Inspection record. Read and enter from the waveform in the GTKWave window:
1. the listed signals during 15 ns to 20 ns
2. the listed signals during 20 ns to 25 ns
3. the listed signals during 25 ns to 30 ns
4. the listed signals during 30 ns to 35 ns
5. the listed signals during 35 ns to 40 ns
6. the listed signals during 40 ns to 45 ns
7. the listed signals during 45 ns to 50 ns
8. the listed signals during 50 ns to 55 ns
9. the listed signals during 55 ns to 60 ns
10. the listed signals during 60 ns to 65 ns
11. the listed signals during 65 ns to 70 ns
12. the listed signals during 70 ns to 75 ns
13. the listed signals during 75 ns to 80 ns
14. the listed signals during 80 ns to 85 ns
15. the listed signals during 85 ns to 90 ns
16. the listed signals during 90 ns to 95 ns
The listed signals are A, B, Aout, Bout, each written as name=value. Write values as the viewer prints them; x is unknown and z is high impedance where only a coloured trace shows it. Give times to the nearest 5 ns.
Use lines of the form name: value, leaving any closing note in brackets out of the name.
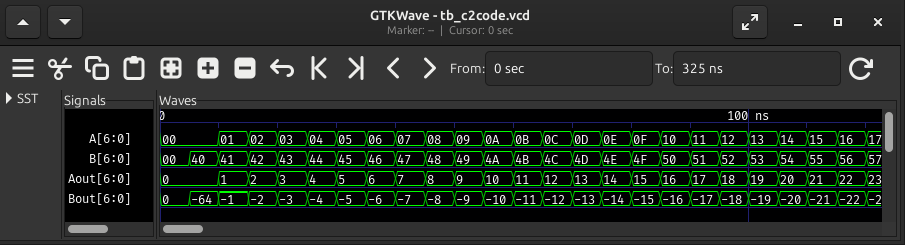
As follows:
the listed signals during 15 ns to 20 ns: A=02, B=42, Aout=2, Bout=-2
the listed signals during 20 ns to 25 ns: A=03, B=43, Aout=3, Bout=-3
the listed signals during 25 ns to 30 ns: A=04, B=44, Aout=4, Bout=-4
the listed signals during 30 ns to 35 ns: A=05, B=45, Aout=5, Bout=-5
the listed signals during 35 ns to 40 ns: A=06, B=46, Aout=6, Bout=-6
the listed signals during 40 ns to 45 ns: A=07, B=47, Aout=7, Bout=-7
the listed signals during 45 ns to 50 ns: A=08, B=48, Aout=8, Bout=-8
the listed signals during 50 ns to 55 ns: A=09, B=49, Aout=9, Bout=-9
the listed signals during 55 ns to 60 ns: A=0A, B=4A, Aout=10, Bout=-10
the listed signals during 60 ns to 65 ns: A=0B, B=4B, Aout=11, Bout=-11
the listed signals during 65 ns to 70 ns: A=0C, B=4C, Aout=12, Bout=-12
the listed signals during 70 ns to 75 ns: A=0D, B=4D, Aout=13, Bout=-13
the listed signals during 75 ns to 80 ns: A=0E, B=4E, Aout=14, Bout=-14
the listed signals during 80 ns to 85 ns: A=0F, B=4F, Aout=15, Bout=-15
the listed signals during 85 ns to 90 ns: A=10, B=50, Aout=16, Bout=-16
the listed signals during 90 ns to 95 ns: A=11, B=51, Aout=17, Bout=-17
